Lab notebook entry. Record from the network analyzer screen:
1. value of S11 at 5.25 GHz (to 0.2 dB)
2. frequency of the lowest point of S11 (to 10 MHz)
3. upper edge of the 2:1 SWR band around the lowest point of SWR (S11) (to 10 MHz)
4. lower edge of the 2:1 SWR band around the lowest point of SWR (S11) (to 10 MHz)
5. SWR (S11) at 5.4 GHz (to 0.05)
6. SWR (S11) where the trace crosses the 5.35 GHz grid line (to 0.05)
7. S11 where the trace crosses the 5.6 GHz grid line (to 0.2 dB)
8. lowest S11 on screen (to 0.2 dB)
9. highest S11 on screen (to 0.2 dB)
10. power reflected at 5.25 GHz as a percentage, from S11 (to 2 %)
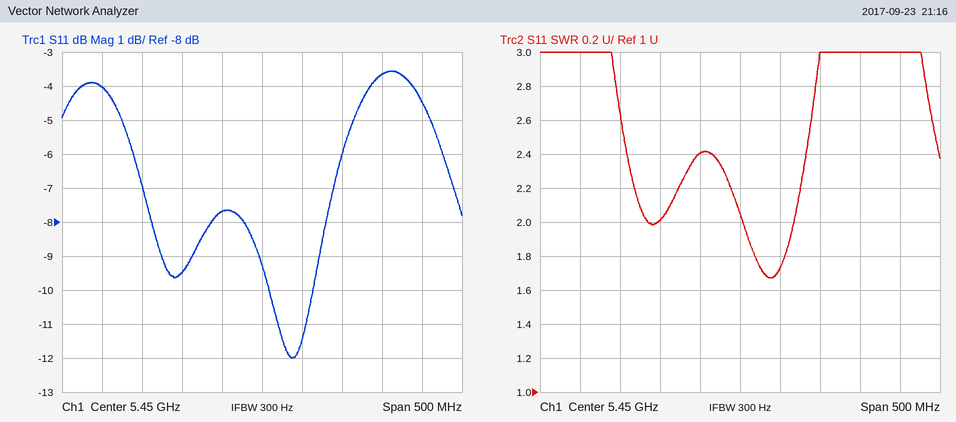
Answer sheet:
-4.0 dB
5.49 GHz
5.52 GHz
5.45 GHz
2.40
2.00
-3.6 dB
-12.0 dB
-3.6 dB
40 %
